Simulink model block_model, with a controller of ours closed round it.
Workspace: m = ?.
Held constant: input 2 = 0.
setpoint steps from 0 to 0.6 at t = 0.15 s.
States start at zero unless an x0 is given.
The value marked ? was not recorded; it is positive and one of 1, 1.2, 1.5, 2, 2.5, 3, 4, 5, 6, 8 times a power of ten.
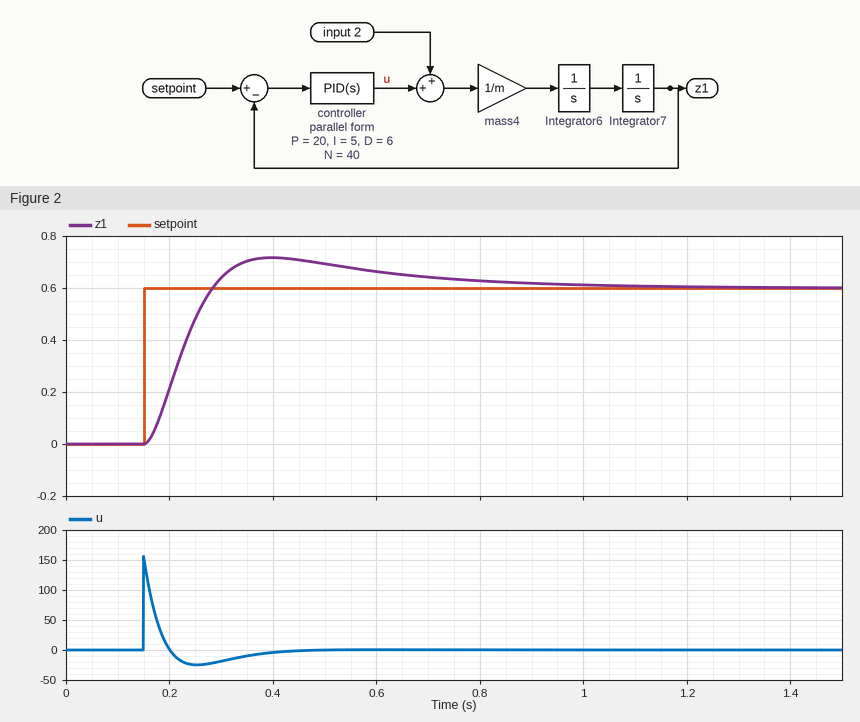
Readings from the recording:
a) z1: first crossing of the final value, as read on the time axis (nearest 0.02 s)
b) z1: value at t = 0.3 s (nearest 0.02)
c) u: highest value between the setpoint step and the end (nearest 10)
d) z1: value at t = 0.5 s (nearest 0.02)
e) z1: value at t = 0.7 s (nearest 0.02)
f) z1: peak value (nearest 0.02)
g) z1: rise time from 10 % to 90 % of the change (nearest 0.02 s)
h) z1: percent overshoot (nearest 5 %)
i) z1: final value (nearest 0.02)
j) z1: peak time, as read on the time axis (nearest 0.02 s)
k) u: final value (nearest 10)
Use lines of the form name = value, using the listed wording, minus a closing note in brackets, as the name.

z1: first crossing of the final value, as read on the time axis = 0.28 s
z1: value at t = 0.3 s = 0.64
u: highest value between the setpoint step and the end = 160
z1: value at t = 0.5 s = 0.70
z1: value at t = 0.7 s = 0.64
z1: peak value = 0.72
z1: rise time from 10 % to 90 % of the change = 0.10 s
z1: percent overshoot = 20 %
z1: final value = 0.60
z1: peak time, as read on the time axis = 0.40 s
u: final value = 0
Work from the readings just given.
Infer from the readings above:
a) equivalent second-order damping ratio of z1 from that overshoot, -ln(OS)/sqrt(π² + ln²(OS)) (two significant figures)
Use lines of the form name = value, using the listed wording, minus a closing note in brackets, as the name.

equivalent second-order damping ratio of z1 from that overshoot, -ln(OS)/sqrt(π² + ln²(OS)) = 0.46
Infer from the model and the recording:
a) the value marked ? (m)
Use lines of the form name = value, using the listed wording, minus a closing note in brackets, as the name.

the value marked ? = 0.5
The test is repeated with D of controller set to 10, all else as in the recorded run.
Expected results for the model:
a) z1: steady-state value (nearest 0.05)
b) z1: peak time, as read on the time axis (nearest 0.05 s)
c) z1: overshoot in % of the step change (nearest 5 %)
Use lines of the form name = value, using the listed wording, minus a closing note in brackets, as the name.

z1: steady-state value = 0.60
z1: peak time, as read on the time axis = 0.30 s
z1: overshoot in % of the step change = 15 %
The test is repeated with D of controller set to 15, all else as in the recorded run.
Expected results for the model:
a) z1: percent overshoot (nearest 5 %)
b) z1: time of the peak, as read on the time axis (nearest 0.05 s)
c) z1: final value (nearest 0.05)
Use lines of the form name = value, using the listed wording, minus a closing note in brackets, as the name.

z1: percent overshoot = 15 %
z1: time of the peak, as read on the time axis = 0.25 s
z1: final value = 0.60
